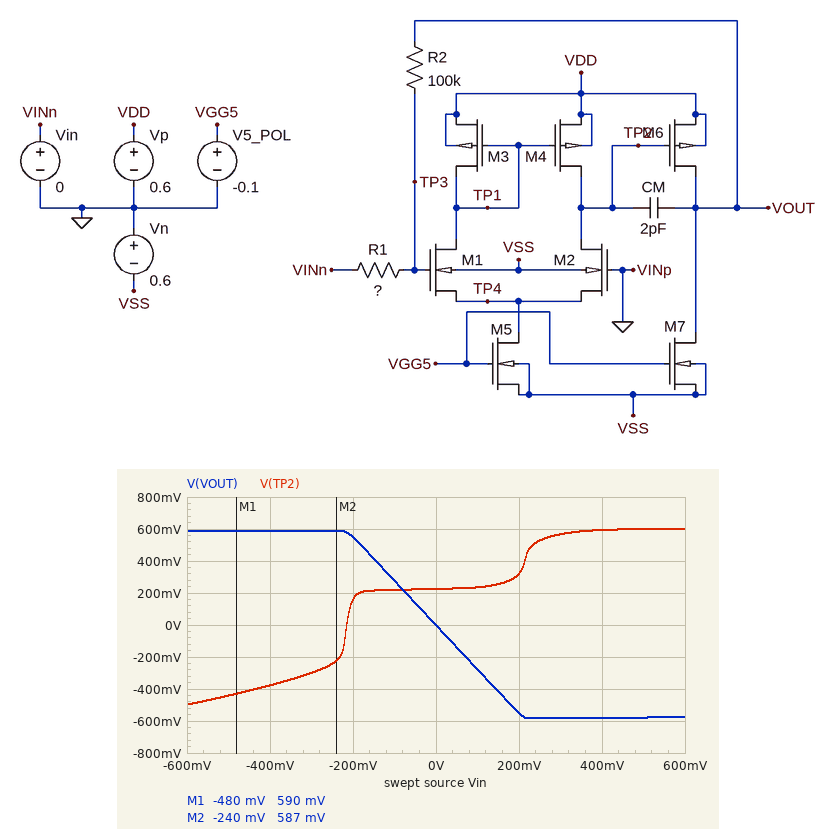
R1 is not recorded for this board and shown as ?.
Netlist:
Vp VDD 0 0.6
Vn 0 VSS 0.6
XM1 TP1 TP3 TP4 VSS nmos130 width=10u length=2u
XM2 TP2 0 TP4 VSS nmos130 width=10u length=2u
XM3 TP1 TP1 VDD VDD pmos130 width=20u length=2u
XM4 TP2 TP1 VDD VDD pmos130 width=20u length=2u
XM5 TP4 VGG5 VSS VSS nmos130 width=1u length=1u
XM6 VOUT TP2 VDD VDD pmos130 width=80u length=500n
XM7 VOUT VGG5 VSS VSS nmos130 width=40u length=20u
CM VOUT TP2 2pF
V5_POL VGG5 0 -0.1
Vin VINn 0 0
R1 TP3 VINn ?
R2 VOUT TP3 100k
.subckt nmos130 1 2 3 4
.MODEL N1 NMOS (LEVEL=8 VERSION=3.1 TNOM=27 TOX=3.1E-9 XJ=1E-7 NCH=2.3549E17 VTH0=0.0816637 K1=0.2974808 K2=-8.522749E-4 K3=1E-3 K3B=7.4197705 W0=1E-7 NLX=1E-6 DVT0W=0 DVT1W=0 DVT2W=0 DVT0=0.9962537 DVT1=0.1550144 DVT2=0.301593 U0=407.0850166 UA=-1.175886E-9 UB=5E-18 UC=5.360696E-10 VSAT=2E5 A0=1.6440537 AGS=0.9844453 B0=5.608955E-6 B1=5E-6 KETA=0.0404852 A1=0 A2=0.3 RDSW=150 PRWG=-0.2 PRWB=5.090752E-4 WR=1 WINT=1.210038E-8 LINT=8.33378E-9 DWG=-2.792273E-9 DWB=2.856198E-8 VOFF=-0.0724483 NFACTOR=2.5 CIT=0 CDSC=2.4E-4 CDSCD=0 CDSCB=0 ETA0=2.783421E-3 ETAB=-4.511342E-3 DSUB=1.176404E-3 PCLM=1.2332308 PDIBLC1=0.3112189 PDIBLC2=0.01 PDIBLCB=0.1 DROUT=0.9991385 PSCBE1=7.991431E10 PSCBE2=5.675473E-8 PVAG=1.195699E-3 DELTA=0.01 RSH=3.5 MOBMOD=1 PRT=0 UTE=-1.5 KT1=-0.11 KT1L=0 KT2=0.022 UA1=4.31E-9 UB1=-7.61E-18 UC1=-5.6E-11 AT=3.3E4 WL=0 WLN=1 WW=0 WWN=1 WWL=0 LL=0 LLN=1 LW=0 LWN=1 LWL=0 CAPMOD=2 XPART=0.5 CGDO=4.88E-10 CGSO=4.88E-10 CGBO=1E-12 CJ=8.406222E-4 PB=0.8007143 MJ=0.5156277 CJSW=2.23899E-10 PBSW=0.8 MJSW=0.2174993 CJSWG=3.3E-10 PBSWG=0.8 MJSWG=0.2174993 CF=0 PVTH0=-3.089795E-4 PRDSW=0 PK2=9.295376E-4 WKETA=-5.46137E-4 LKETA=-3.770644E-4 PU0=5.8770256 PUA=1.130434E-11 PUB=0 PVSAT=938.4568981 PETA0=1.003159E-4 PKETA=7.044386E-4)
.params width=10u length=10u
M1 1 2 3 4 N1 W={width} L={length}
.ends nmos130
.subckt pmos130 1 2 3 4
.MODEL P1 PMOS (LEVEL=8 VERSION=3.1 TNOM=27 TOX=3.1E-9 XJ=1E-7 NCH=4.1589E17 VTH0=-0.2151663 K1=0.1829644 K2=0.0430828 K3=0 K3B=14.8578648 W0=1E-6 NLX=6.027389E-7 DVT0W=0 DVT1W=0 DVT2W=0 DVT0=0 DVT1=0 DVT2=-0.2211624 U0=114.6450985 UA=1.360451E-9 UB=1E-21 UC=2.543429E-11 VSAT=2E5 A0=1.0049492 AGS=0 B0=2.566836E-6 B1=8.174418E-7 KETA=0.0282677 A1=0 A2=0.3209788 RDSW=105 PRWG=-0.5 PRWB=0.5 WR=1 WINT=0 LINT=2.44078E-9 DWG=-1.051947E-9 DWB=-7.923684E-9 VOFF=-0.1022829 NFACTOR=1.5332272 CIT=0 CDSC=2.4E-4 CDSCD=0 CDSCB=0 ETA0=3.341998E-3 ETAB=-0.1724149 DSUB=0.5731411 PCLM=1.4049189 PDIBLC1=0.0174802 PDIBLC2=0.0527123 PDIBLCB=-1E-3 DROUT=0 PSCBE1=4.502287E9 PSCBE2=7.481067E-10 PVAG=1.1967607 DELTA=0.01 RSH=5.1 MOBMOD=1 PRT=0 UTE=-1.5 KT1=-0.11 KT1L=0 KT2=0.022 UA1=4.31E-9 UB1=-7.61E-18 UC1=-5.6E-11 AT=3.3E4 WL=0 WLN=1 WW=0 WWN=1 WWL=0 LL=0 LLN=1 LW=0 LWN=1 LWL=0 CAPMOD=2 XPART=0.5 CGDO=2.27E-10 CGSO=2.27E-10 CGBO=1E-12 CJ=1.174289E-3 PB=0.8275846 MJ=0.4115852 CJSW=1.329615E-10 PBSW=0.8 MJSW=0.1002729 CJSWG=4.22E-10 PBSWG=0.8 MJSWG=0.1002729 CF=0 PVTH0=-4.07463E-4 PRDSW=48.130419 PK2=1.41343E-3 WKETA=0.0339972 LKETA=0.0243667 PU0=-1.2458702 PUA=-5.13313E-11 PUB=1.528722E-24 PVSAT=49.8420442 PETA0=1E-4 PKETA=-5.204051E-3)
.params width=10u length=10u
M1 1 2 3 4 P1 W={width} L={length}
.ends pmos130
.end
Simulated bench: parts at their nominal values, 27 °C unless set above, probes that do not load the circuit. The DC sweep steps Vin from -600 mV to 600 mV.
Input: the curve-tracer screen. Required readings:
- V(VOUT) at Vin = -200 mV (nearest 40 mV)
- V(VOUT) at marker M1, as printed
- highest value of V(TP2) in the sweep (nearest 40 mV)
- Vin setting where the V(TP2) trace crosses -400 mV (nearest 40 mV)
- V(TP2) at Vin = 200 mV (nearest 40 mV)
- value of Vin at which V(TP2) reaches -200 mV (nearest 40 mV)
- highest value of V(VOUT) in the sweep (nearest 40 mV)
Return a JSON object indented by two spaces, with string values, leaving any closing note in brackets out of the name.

{
  "V(VOUT) at Vin = -200 mV": "560 mV",
  "V(VOUT) at marker M1, as printed": "590 mV",
  "highest value of V(TP2) in the sweep": "600 mV",
  "Vin setting where the V(TP2) trace crosses -400 mV": "-440 mV",
  "V(TP2) at Vin = 200 mV": "320 mV",
  "value of Vin at which V(TP2) reaches -200 mV": "-240 mV",
  "highest value of V(VOUT) in the sweep": "600 mV"
}
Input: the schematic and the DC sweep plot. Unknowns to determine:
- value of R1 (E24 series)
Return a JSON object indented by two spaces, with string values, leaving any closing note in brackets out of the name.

{
  "value of R1": "36 kΩ"
}
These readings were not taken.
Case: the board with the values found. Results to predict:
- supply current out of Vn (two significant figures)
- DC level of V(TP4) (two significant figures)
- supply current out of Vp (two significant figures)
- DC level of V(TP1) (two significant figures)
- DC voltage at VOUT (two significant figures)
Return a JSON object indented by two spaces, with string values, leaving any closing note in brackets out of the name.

{
  "supply current out of Vn": "95 µA",
  "DC level of V(TP4)": "-280 mV",
  "supply current out of Vp": "95 µA",
  "DC level of V(TP1)": "240 mV",
  "DC voltage at VOUT": "-1.0 mV"
}
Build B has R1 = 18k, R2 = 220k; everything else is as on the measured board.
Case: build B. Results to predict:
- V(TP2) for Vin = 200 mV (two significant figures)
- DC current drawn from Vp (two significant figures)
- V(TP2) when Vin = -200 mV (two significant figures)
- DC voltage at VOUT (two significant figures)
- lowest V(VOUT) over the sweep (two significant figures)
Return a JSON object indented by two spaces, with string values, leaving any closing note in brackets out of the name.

{
  "V(TP2) for Vin = 200 mV": "590 mV",
  "DC current drawn from Vp": "95 µA",
  "V(TP2) when Vin = -200 mV": "-380 mV",
  "DC voltage at VOUT": "-3.5 mV",
  "lowest V(VOUT) over the sweep": "-590 mV"
}
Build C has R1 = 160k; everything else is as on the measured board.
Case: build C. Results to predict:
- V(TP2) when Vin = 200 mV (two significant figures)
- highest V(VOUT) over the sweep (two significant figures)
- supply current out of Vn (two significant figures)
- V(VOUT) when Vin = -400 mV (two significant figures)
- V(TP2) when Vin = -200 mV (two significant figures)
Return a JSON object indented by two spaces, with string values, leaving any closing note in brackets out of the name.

{
  "V(TP2) when Vin = 200 mV": "230 mV",
  "highest V(VOUT) over the sweep": "370 mV",
  "supply current out of Vn": "95 µA",
  "V(VOUT) when Vin = -400 mV": "250 mV",
  "V(TP2) when Vin = -200 mV": "220 mV"
}
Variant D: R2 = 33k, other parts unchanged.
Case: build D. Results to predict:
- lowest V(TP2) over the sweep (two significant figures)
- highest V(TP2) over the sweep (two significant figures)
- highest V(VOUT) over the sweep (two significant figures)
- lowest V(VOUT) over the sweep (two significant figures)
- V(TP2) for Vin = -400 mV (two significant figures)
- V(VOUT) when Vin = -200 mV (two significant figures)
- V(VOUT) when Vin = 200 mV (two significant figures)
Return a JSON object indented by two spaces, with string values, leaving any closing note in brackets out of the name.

{
  "lowest V(TP2) over the sweep": "150 mV",
  "highest V(TP2) over the sweep": "380 mV",
  "highest V(VOUT) over the sweep": "550 mV",
  "lowest V(VOUT) over the sweep": "-540 mV",
  "V(TP2) for Vin = -400 mV": "210 mV",
  "V(VOUT) when Vin = -200 mV": "180 mV",
  "V(VOUT) when Vin = 200 mV": "-180 mV"
}
